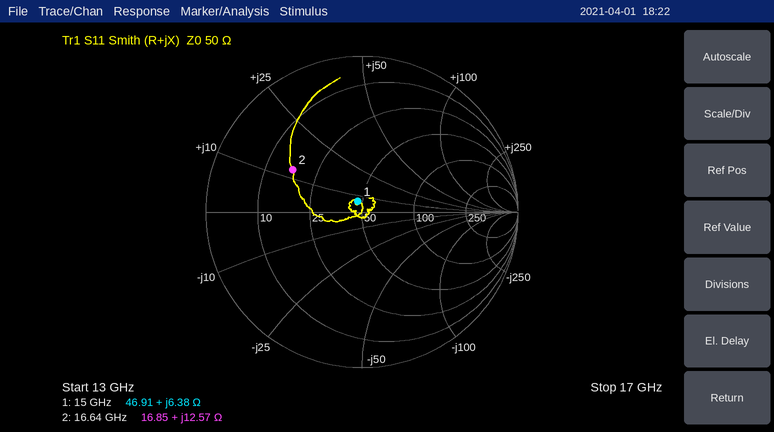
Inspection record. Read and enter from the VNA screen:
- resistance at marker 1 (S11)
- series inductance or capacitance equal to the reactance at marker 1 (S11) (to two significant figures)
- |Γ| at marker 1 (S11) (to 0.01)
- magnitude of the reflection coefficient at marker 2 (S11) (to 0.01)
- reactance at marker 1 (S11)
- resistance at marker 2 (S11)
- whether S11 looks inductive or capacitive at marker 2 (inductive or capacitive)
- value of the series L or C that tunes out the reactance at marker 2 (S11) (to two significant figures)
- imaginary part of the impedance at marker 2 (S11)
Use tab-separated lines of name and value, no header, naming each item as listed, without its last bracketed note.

resistance at marker 1	46.91 Ω
series inductance or capacitance equal to the reactance at marker 1 (S11)	68 pH
|Γ| at marker 1 (S11)	0.07
magnitude of the reflection coefficient at marker 2 (S11)	0.52
reactance at marker 1	+6.38 Ω
resistance at marker 2	16.85 Ω
whether S11 looks inductive or capacitive at marker 2	inductive
value of the series L or C that tunes out the reactance at marker 2 (S11)	760 fF
imaginary part of the impedance at marker 2	+12.57 Ω
